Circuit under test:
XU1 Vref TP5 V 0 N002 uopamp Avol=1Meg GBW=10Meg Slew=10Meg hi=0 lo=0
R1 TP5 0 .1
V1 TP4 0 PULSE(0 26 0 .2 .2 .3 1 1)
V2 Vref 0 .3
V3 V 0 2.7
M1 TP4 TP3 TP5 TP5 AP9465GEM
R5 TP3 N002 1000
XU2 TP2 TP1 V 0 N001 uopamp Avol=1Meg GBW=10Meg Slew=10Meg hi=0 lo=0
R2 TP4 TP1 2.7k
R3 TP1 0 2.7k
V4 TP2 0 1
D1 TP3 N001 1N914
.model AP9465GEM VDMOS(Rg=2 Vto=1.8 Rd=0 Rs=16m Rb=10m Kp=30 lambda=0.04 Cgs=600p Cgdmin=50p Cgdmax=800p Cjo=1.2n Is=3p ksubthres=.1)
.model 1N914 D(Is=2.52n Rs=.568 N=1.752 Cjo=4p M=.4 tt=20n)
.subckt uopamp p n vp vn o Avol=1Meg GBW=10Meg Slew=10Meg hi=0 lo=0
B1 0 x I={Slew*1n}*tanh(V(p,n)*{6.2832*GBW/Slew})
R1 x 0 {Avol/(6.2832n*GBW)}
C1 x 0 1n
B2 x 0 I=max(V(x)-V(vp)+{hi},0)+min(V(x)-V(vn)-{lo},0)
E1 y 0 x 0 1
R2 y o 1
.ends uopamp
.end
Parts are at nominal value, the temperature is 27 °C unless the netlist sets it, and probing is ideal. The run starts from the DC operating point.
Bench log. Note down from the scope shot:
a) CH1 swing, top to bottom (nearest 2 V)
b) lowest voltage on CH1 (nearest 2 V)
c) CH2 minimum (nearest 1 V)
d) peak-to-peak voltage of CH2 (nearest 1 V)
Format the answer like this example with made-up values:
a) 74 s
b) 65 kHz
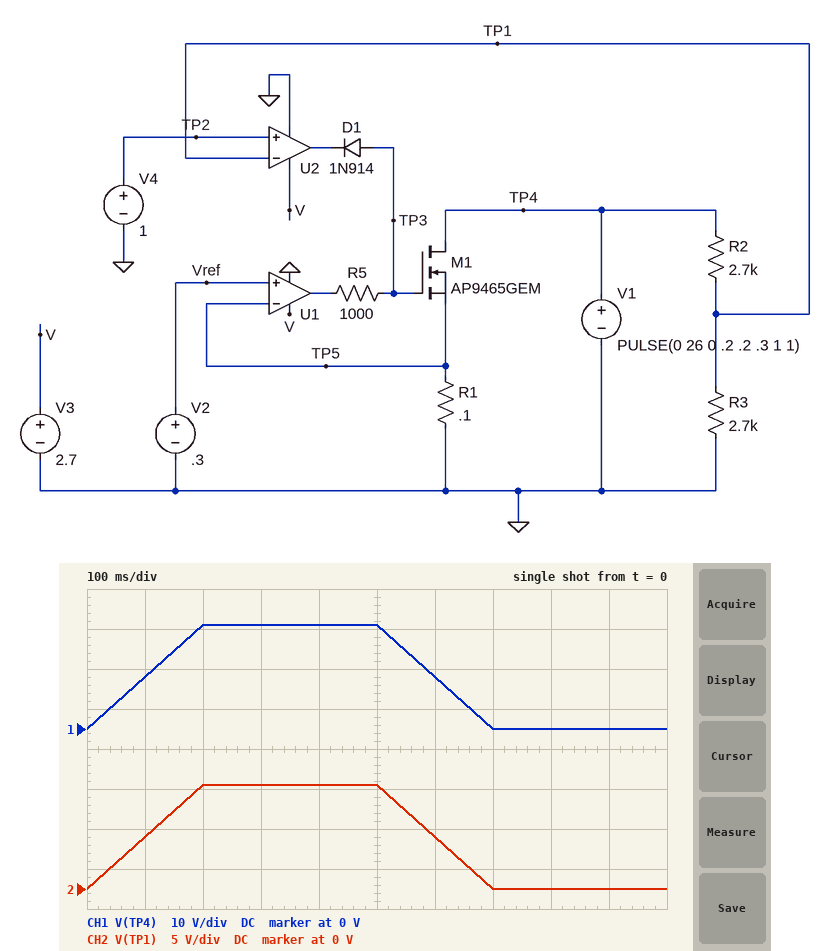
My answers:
a) 26 V
b) 0 V
c) 0 V
d) 13 V
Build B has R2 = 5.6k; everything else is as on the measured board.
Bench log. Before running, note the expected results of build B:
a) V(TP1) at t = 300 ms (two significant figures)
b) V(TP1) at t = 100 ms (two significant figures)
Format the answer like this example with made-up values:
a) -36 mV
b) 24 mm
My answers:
a) 8.5 V
b) 4.2 V
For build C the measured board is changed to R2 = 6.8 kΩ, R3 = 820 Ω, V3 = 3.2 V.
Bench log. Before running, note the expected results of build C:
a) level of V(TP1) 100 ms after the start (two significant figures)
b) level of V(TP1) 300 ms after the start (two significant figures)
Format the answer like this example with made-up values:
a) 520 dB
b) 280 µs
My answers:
a) 1.4 V
b) 2.8 V
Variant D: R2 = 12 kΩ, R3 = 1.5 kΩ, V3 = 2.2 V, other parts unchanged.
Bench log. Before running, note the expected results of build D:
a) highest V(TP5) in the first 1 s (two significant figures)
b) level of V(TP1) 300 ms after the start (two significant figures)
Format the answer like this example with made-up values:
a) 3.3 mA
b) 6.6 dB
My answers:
a) 140 mV
b) 2.9 V
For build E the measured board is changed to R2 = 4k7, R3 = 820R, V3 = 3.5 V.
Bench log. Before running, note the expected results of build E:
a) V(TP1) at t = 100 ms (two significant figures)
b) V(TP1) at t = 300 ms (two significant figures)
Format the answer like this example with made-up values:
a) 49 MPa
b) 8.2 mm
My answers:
a) 1.9 V
b) 3.9 V
